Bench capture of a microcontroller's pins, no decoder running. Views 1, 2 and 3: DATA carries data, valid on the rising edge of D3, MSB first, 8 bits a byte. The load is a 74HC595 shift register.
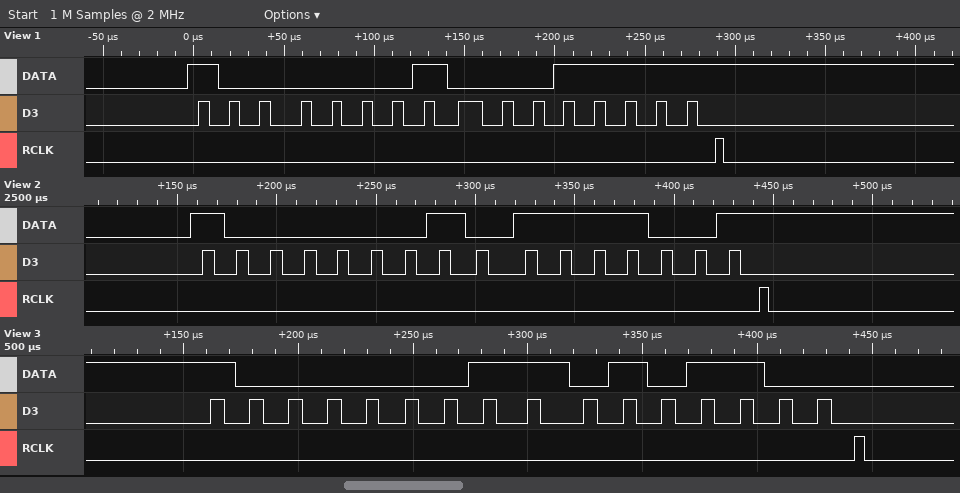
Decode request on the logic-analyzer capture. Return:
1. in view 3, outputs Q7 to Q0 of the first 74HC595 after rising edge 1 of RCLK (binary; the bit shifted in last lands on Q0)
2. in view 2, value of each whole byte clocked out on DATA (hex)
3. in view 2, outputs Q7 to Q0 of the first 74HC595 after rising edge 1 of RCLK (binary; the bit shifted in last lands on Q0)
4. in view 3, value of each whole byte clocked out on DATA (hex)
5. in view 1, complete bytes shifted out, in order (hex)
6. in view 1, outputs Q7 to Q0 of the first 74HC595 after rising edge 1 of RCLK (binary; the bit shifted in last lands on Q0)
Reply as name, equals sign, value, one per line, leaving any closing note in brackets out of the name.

in view 3, outputs Q7 to Q0 of the first 74HC595 after rising edge 1 of RCLK = 10101100
in view 2, value of each whole byte clocked out on DATA = 81 79
in view 2, outputs Q7 to Q0 of the first 74HC595 after rising edge 1 of RCLK = 01111001
in view 3, value of each whole byte clocked out on DATA = 0x81 0xAC
in view 1, complete bytes shifted out, in order = 81 1F
in view 1, outputs Q7 to Q0 of the first 74HC595 after rising edge 1 of RCLK = 00011111
